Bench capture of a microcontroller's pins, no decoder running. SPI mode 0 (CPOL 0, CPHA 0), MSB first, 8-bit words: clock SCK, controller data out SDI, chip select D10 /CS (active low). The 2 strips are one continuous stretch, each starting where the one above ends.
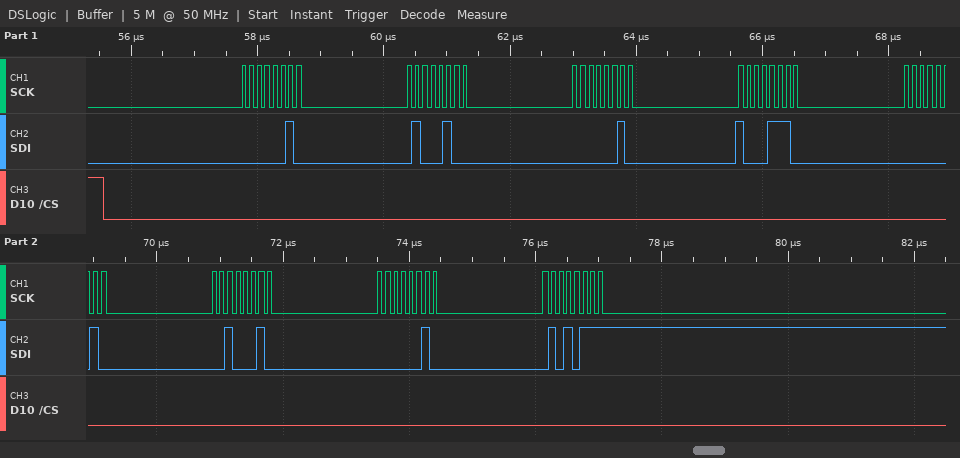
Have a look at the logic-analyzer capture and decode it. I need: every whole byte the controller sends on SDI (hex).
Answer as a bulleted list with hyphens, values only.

- 02 44 02 8E 02 22 02 57
